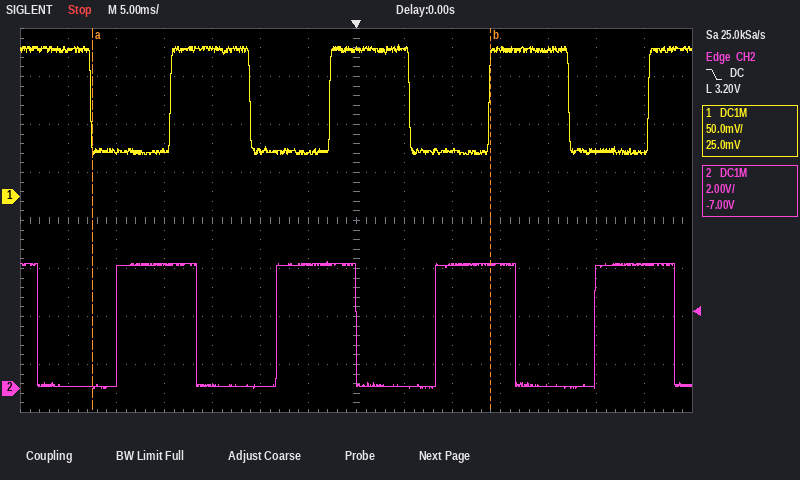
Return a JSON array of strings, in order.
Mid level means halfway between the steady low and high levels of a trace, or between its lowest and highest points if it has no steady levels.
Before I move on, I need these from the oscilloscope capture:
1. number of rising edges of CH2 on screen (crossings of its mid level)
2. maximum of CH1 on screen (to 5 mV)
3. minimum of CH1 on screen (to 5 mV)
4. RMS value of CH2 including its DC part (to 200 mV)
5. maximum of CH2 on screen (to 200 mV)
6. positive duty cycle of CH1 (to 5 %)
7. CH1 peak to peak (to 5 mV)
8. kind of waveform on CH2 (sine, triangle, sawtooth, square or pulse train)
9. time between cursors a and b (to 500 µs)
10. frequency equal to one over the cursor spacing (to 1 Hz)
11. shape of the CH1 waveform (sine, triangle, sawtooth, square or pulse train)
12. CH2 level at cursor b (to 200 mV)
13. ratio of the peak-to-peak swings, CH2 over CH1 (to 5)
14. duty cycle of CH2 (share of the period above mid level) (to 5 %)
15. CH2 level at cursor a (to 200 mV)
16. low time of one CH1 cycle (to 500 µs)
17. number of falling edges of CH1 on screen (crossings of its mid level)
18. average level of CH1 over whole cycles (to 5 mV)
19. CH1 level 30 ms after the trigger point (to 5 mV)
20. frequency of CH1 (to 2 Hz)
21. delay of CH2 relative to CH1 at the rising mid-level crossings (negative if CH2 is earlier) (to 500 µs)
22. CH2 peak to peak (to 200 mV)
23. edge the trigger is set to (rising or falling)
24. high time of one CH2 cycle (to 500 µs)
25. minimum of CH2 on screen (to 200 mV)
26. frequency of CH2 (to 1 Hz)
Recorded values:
["4", "160 mV", "45 mV", "3.6 V", "5.2 V", "50 %", "115 mV", "square", "41.5 ms", "24 Hz", "square", "5.2 V", "45", "50 %", "0.0 V", "8.5 ms", "4", "100 mV", "45 mV", "60 Hz", "-5.5 ms", "5.2 V", "falling", "8.5 ms", "0.0 V", "60 Hz"]
